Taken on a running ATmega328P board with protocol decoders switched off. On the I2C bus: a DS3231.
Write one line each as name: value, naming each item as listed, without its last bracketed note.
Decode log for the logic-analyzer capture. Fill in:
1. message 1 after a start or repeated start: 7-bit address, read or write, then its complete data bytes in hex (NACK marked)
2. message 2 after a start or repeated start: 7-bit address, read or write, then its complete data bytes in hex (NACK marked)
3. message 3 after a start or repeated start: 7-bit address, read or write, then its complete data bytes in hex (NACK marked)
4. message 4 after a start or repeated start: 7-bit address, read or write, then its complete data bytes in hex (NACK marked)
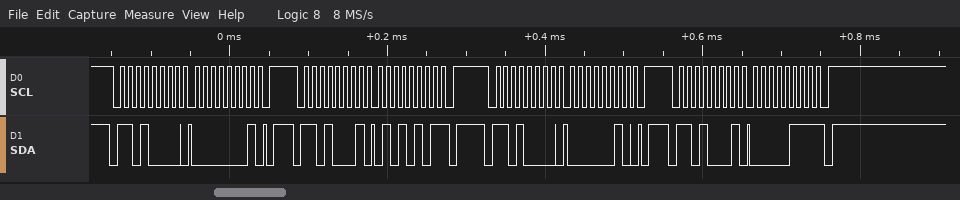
message 1 after a start or repeated start: 7-bit address, read or write, then its complete data bytes in hex: 0x68 write: 01
message 2 after a start or repeated start: 7-bit address, read or write, then its complete data bytes in hex: 0x68 read: 55 NACK
message 3 after a start or repeated start: 7-bit address, read or write, then its complete data bytes in hex: 0x68 write: 02
message 4 after a start or repeated start: 7-bit address, read or write, then its complete data bytes in hex: 0x68 read: 07 NACK
